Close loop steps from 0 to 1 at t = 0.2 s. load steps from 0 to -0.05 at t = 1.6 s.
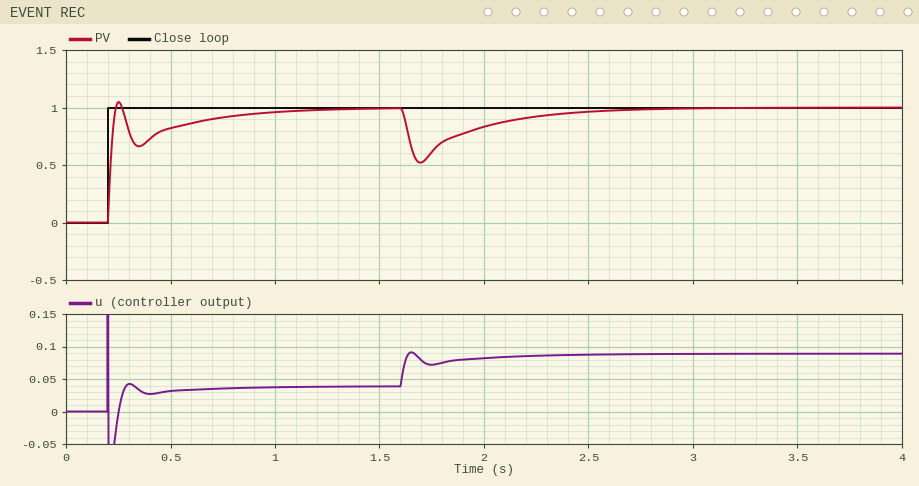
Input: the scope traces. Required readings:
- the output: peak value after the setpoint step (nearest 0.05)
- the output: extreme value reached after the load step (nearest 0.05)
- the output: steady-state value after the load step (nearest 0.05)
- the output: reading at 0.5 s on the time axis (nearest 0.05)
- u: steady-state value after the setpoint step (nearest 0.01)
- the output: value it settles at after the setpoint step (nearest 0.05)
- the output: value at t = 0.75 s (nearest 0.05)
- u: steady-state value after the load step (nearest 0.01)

1.05
0.50
1.00
0.80
0.04
1.00
0.90
0.09
